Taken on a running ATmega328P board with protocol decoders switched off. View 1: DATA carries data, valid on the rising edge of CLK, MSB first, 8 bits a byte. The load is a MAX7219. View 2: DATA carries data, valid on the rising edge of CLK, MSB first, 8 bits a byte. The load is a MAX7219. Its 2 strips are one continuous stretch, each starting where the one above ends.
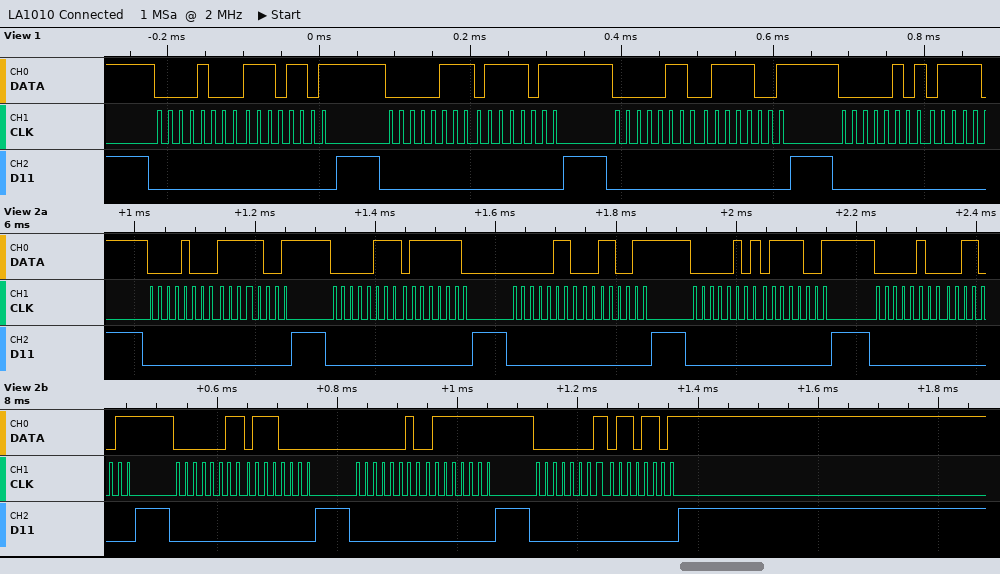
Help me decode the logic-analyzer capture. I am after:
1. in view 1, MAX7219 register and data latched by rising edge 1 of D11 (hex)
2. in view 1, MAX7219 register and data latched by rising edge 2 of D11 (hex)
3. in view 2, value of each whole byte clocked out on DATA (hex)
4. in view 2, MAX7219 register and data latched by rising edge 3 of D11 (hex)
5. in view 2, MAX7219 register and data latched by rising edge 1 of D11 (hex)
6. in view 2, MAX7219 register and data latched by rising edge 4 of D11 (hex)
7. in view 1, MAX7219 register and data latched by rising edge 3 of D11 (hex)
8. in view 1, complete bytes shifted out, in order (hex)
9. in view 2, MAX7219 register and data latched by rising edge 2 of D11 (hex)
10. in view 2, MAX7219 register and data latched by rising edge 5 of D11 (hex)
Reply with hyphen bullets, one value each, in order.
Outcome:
- register 0x8, data 0xED
- register 0x7, data 0x7B
- 08 F9 07 7E 06 33 05 79 04 33 03 70 02 7F 01 6D
- register 0x6, data 0x33
- register 0x8, data 0xF9
- register 0x5, data 0x79
- register 0x6, data 0x79
- 08 ED 07 7B 06 79 05
- register 0x7, data 0x7E
- register 0x4, data 0x33
